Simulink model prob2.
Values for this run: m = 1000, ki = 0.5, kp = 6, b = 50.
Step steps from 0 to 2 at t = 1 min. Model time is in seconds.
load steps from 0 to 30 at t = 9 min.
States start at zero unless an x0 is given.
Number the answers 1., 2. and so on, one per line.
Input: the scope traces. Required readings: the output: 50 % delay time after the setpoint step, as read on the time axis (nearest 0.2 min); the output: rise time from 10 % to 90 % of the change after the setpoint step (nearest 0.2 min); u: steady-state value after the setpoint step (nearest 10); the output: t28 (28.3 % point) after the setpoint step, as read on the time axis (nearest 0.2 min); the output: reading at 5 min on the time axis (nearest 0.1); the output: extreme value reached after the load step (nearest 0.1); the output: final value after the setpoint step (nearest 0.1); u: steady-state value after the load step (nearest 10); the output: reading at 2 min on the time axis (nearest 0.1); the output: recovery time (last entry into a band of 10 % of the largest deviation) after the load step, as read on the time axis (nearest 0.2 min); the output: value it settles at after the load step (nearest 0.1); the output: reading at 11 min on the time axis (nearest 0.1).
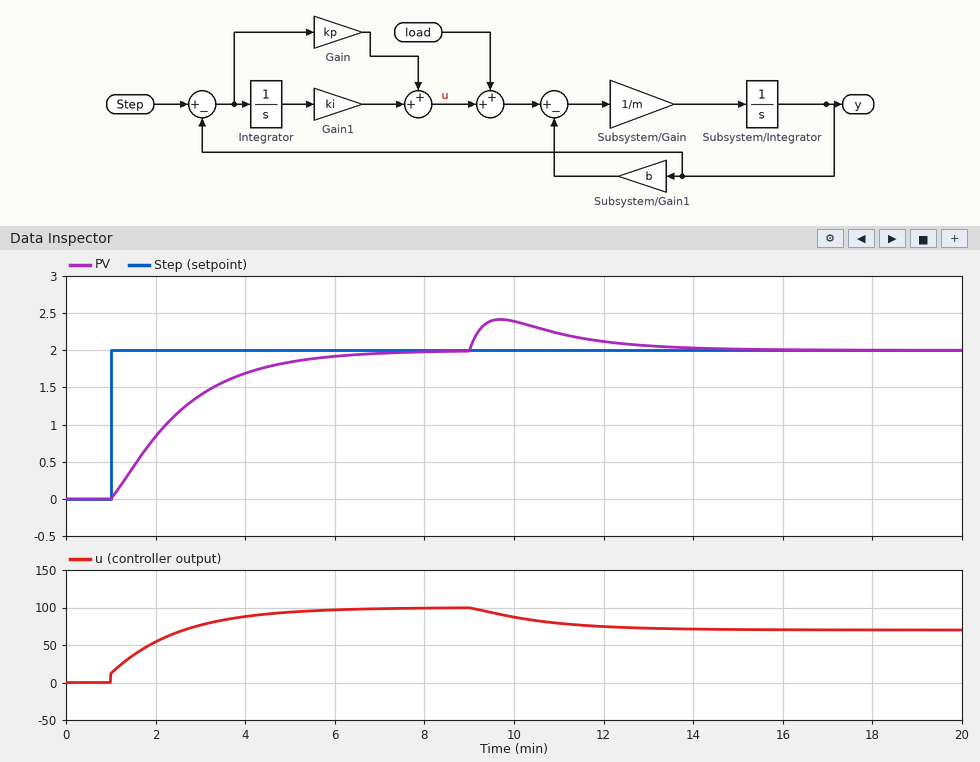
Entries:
1. 2.2 min
2. 3.4 min
3. 100
4. 1.6 min
5. 1.8
6. 2.4
7. 2.0
8. 70
9. 0.8
10. 13.6 min
11. 2.0
12. 2.2
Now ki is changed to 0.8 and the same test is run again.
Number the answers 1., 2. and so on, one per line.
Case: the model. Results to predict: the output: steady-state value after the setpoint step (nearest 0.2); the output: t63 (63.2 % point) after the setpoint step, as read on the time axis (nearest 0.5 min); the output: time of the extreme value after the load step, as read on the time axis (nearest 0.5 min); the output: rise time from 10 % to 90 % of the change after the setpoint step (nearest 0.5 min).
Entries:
1. 2.0
2. 2.0 min
3. 9.5 min
4. 2.0 min
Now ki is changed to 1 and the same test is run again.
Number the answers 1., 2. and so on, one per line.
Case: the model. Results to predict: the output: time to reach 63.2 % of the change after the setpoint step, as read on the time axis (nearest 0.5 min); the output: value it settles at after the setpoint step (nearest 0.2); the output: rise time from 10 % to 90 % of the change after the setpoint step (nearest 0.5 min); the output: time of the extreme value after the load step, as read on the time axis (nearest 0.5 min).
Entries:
1. 2.0 min
2. 2.0
3. 1.5 min
4. 9.5 min
